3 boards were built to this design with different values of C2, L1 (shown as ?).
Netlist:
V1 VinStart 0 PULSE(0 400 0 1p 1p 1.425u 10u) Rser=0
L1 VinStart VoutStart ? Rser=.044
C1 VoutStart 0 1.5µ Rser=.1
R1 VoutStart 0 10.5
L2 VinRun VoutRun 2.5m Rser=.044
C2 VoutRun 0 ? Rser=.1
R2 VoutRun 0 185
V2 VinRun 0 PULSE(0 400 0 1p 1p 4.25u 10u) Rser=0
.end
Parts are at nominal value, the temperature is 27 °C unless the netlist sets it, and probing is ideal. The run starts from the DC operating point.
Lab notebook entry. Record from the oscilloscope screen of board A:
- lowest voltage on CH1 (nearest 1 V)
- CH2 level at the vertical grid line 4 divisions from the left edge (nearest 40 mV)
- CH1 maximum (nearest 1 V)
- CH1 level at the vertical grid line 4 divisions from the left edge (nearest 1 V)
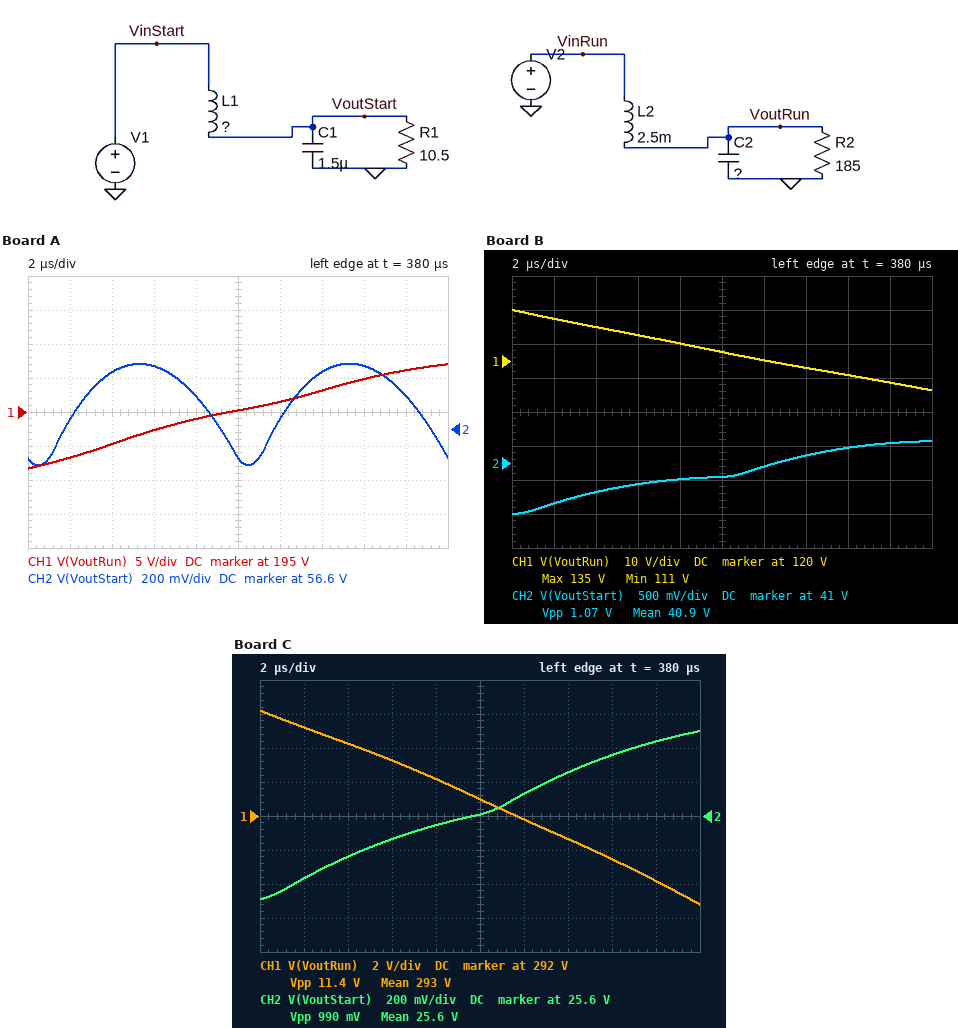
187 V
56.80 V
202 V
194 V
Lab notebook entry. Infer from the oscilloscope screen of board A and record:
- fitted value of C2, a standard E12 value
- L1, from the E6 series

820 nF
680 µH
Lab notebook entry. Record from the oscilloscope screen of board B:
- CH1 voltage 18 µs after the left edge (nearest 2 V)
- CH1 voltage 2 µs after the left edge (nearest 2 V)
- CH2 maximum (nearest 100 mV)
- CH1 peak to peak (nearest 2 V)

114 V
132 V
41.3 V
24 V
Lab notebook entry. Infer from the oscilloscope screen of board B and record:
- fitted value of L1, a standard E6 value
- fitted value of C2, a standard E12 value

3.3 mH
2.2 µF
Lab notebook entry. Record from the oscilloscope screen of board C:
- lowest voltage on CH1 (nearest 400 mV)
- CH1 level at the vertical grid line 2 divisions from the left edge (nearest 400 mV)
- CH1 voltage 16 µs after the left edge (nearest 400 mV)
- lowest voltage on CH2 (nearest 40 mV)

286.8 V
296.4 V
289.6 V
25.12 V
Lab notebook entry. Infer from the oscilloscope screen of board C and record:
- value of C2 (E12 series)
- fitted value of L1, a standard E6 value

4.7 µF
6.8 mH
